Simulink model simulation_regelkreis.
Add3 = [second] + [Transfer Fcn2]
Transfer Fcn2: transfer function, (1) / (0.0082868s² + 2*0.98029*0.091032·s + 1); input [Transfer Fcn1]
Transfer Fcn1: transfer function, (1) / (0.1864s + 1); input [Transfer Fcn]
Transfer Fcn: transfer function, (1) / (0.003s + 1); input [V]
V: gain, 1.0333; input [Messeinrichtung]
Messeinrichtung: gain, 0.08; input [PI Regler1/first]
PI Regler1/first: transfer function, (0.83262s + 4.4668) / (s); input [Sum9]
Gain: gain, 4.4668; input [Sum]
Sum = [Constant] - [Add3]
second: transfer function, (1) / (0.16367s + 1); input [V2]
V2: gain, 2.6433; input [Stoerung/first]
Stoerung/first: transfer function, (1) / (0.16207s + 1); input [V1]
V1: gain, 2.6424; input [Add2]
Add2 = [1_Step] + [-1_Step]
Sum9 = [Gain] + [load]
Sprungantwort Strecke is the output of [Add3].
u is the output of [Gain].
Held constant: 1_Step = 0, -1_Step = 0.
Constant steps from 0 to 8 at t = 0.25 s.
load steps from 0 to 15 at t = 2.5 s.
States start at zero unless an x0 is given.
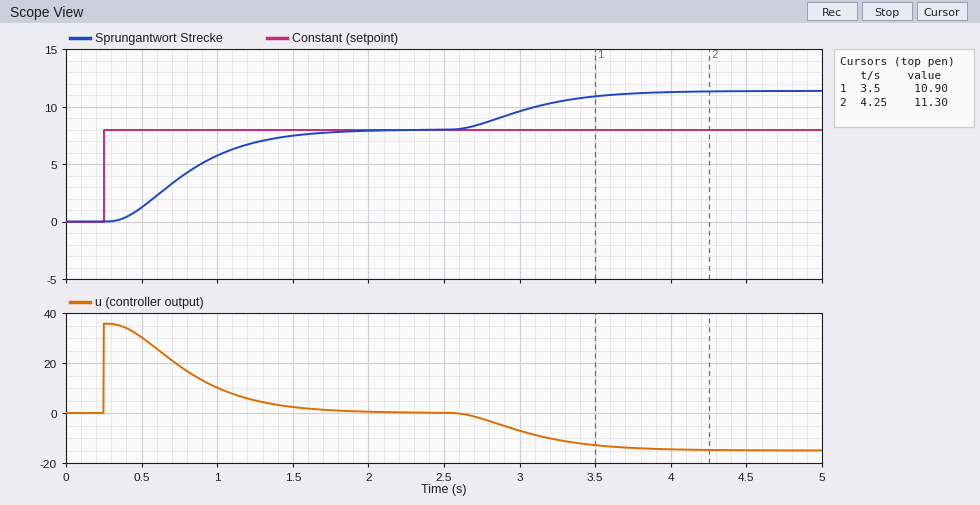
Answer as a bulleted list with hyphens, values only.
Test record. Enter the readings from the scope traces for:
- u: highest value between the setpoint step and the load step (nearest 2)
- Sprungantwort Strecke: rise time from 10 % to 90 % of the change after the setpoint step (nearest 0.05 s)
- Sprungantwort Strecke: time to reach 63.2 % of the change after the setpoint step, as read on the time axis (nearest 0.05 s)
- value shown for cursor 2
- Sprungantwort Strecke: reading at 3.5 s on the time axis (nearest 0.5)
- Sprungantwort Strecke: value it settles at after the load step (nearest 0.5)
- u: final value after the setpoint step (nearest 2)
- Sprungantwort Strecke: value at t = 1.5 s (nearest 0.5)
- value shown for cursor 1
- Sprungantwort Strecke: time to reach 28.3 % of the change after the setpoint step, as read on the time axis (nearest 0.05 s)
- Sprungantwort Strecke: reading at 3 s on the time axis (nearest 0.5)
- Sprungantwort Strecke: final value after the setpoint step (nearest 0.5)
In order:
- 36
- 0.90 s
- 0.90 s
- 11.30
- 11.0
- 11.5
- 0
- 7.5
- 10.90
- 0.60 s
- 9.5
- 8.0
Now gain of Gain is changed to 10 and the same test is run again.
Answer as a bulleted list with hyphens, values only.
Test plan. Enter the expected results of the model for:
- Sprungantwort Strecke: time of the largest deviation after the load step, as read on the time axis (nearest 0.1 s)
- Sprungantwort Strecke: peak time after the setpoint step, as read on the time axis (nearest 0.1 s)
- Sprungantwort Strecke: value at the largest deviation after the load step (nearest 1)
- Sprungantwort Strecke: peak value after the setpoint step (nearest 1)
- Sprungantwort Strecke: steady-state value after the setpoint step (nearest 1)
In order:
- 3.3 s
- 1.0 s
- 10
- 9
- 8
